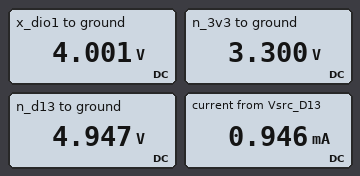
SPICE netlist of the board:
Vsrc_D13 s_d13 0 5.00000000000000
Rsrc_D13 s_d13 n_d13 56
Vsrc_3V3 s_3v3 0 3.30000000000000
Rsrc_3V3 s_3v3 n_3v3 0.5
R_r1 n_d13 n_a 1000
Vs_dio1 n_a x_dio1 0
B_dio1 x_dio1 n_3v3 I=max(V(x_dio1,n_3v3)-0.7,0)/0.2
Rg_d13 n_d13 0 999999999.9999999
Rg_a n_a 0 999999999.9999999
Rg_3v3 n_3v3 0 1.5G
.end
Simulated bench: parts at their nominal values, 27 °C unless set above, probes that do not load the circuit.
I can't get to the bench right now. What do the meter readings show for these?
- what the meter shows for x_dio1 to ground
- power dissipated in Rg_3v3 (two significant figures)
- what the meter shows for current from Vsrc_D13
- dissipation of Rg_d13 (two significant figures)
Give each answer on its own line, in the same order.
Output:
4.001 V
7.3 nW
0.946 mA
24 nW
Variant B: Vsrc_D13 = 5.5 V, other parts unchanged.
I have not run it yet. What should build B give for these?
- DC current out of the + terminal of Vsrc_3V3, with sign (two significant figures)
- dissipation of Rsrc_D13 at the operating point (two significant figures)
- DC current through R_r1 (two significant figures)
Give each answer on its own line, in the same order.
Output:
-1.4 mA
110 µW
1.4 mA
